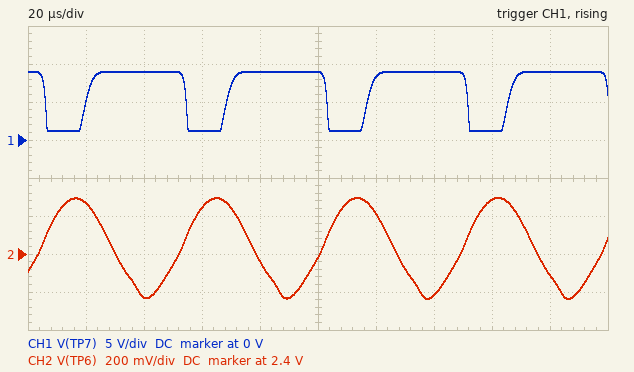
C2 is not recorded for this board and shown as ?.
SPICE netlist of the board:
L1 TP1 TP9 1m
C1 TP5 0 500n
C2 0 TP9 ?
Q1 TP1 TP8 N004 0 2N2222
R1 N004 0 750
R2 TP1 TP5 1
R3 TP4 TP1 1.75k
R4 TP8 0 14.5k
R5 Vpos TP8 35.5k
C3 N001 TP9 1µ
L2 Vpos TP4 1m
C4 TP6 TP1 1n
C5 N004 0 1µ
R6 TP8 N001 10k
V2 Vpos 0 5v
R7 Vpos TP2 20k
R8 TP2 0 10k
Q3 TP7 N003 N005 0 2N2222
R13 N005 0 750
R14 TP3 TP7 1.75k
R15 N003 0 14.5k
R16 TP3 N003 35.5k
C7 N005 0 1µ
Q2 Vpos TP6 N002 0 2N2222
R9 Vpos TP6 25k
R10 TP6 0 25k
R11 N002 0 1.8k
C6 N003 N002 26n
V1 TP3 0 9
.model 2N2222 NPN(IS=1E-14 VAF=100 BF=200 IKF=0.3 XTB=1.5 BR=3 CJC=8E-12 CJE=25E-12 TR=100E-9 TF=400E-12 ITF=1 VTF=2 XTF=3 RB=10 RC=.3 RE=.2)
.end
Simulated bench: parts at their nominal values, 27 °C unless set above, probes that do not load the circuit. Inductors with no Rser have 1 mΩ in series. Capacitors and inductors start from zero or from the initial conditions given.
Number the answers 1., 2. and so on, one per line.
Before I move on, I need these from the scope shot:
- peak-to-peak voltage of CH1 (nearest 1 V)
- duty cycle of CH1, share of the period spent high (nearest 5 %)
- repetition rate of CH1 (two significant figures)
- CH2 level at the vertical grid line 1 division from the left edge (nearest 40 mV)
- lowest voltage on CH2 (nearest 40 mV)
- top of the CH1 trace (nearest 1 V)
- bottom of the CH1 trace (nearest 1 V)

1. 8 V
2. 70 %
3. 21 kHz
4. 2.68 V
5. 2.16 V
6. 9 V
7. 1 V
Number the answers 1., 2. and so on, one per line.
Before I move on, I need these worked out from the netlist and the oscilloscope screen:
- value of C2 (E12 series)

1. 68 nF
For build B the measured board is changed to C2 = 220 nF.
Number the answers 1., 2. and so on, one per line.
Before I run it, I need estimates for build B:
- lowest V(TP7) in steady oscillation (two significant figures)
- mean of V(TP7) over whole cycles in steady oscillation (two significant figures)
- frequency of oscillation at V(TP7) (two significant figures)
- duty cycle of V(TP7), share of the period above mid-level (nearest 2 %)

1. 1.0 V
2. 6.9 V
3. 13 kHz
4. 74 %
